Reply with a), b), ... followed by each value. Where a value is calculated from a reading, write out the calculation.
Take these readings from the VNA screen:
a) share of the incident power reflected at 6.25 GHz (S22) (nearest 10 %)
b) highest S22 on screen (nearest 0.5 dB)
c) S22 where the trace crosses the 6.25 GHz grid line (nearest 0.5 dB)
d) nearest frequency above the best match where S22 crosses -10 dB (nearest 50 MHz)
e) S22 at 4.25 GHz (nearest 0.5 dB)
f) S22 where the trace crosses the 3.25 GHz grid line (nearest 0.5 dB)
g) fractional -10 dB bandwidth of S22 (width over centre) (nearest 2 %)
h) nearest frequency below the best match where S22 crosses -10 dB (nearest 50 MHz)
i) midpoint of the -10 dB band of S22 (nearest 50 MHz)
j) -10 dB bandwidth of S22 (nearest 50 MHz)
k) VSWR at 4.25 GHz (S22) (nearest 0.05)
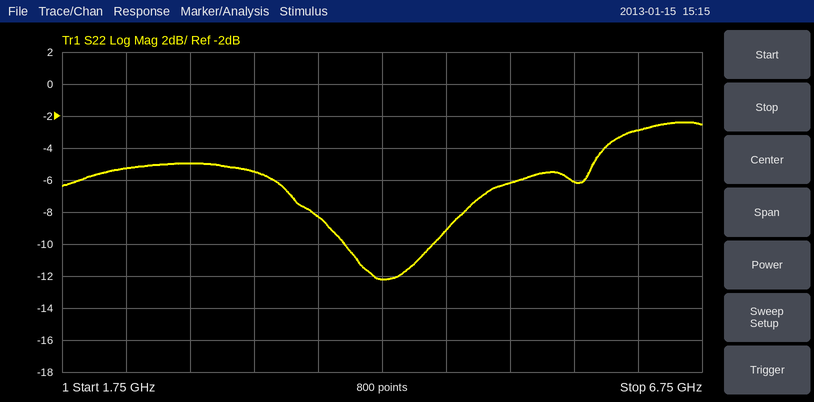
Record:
a) 10^(-3/10) ≈ 50 %
b) -2.5 dB
c) -3.0 dB
d) 4.65 GHz
e) -12.0 dB
f) -5.5 dB
g) 700 MHz / 4.3 GHz ≈ 16 %
h) 3.95 GHz
i) 4.30 GHz
j) 4.65 GHz − 3.95 GHz = 700 MHz
k) |Γ| = 10^(-12/20) = 0.2512; VSWR = (1 + 0.2512)/(1 − 0.2512) ≈ 1.67, so 1.65 to the nearest 0.05
